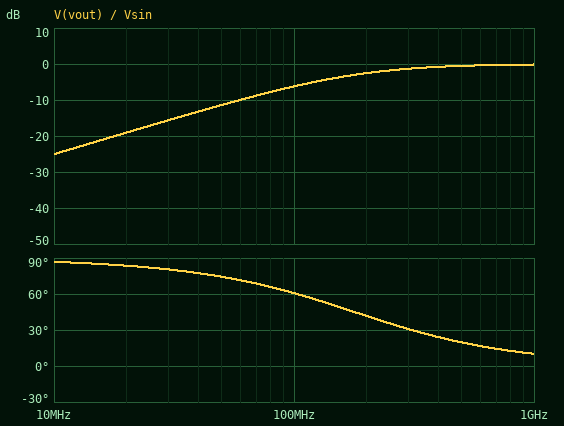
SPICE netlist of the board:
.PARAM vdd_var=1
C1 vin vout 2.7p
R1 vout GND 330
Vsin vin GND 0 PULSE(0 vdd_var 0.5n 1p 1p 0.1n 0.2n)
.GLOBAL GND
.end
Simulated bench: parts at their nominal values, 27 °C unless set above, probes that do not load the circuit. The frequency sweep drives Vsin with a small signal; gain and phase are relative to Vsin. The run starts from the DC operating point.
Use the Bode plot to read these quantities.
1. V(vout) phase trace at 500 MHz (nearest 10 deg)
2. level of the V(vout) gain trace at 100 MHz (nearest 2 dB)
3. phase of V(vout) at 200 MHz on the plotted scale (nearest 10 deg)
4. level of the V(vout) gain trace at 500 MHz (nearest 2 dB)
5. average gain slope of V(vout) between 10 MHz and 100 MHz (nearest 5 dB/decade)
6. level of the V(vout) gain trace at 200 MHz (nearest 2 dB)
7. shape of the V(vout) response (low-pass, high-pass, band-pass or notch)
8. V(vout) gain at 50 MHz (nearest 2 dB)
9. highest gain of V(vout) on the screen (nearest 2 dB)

20 deg
-6 dB
40 deg
0 dB
20 dB/decade
-2 dB
high-pass
-12 dB
0 dB
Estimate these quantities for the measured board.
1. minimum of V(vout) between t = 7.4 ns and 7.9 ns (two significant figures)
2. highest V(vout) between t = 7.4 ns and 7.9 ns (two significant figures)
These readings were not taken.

-530 mV
520 mV
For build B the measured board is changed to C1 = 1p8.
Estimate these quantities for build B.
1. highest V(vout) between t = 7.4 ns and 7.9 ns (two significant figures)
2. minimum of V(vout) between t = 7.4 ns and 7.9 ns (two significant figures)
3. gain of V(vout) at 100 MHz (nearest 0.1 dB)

540 mV
-550 mV
-9.1 dB
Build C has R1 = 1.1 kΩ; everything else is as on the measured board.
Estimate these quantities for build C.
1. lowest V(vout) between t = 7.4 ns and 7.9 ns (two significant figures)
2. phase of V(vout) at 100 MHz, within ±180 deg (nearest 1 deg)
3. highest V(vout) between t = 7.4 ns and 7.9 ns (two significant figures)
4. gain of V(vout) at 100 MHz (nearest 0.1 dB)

-470 mV
28 deg
550 mV
-1.1 dB
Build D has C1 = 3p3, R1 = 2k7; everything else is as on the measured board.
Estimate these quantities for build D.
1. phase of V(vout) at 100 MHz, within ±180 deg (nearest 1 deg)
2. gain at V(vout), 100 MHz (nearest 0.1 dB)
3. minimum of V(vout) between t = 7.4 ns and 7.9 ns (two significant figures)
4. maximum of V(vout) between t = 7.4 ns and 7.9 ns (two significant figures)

10 deg
-0.1 dB
-290 mV
730 mV
